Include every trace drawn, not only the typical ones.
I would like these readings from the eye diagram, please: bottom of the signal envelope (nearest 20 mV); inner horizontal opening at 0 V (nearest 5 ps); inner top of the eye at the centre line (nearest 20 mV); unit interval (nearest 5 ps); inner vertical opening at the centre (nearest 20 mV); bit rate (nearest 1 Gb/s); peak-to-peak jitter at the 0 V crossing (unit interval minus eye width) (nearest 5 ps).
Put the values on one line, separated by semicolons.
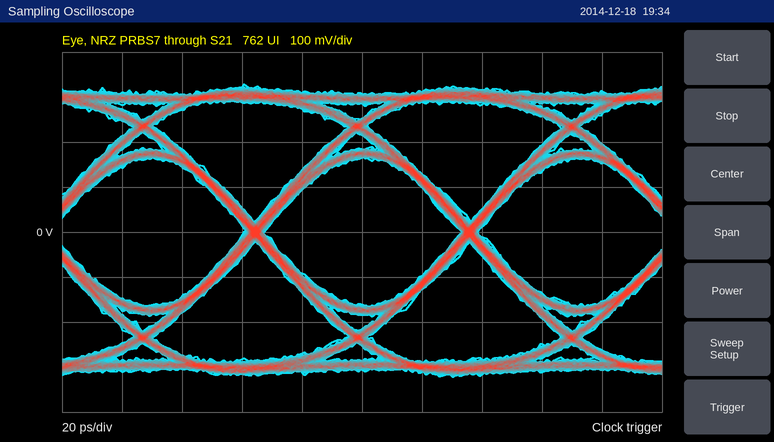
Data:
-320 mV; 65 ps; 160 mV; 70 ps; 320 mV; 14 Gb/s; 5 ps
